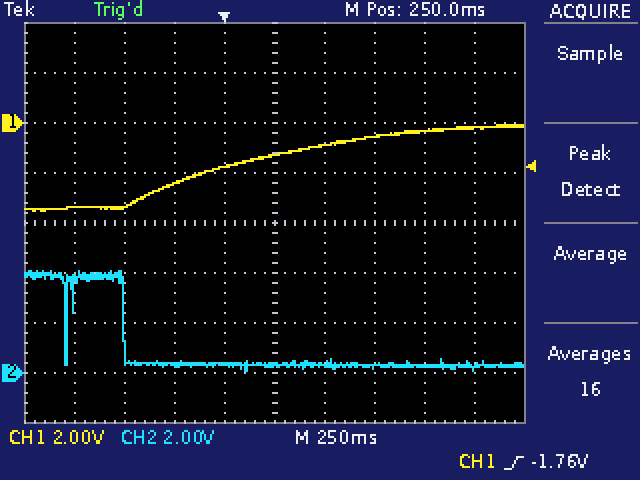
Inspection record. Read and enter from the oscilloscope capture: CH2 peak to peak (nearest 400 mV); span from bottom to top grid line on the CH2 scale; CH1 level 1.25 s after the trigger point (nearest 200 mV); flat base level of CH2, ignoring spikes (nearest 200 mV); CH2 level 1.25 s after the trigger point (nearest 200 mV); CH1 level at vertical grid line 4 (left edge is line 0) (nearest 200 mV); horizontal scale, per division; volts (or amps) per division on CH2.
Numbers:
4.0 V
16 V
-200 mV
400 mV
200 mV
-1.8 V
250 ms
2 V
